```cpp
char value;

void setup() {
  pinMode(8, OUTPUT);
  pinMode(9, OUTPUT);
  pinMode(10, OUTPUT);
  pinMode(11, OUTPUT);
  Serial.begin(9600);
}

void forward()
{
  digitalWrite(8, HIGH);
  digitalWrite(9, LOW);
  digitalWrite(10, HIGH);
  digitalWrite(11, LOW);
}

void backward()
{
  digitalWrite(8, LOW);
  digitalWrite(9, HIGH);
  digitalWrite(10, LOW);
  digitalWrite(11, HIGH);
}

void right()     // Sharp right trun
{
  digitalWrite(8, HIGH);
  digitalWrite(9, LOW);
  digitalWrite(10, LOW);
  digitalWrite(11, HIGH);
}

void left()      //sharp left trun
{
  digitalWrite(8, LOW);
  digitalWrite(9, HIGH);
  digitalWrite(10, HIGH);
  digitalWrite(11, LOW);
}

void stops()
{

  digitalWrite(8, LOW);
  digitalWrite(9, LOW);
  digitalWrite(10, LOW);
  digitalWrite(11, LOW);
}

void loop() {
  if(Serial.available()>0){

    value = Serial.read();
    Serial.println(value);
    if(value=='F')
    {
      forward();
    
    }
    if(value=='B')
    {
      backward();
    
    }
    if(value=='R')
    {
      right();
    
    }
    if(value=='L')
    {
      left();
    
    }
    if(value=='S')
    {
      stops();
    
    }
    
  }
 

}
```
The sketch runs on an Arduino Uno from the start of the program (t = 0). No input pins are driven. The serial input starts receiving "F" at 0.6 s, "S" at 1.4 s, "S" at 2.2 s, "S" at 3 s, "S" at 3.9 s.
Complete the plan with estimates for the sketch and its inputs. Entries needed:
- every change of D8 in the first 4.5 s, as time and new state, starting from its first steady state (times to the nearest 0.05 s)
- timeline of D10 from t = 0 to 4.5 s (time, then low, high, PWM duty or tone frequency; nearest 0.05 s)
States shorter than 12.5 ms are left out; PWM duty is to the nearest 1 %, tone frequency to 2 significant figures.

0 s low; 0.6 s high; 1.4 s low
0 s low; 0.6 s high; 1.4 s low
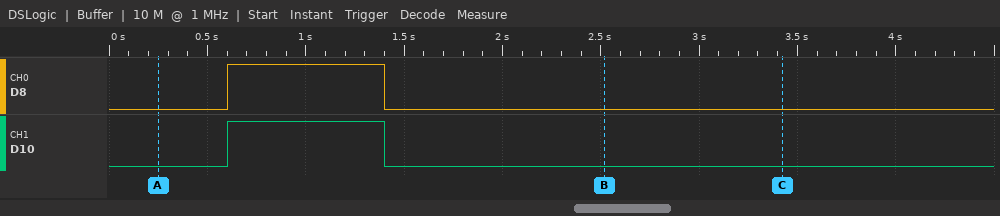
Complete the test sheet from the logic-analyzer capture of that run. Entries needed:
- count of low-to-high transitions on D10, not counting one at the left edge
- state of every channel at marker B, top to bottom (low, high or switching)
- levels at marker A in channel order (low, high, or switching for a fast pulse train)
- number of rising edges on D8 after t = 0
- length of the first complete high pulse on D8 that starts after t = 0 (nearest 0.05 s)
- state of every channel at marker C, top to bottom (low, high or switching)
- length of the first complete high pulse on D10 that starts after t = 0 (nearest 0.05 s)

1
D8 low, D10 low
D8 low, D10 low
1
0.80 s
D8 low, D10 low
0.80 s
